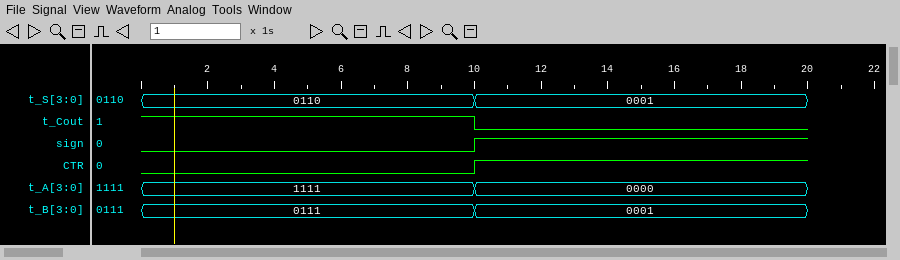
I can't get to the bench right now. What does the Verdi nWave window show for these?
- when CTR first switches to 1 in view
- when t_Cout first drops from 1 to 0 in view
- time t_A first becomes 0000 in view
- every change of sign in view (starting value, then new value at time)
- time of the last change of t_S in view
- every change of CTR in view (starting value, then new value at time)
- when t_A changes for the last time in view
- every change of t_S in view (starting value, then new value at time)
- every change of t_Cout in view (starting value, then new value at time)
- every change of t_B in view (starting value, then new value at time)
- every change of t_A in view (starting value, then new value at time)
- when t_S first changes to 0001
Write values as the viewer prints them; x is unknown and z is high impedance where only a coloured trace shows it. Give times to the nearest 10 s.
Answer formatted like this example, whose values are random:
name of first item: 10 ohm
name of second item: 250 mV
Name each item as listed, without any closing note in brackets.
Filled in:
when CTR first switches to 1 in view: 10 s
when t_Cout first drops from 1 to 0 in view: 10 s
time t_A first becomes 0000 in view: 10 s
every change of sign in view: 0, 1 at 10 s
time of the last change of t_S in view: 10 s
every change of CTR in view: 0, 1 at 10 s
when t_A changes for the last time in view: 10 s
every change of t_S in view: 0110, 0001 at 10 s
every change of t_Cout in view: 1, 0 at 10 s
every change of t_B in view: 0111, 0001 at 10 s
every change of t_A in view: 1111, 0000 at 10 s
when t_S first changes to 0001: 10 s
